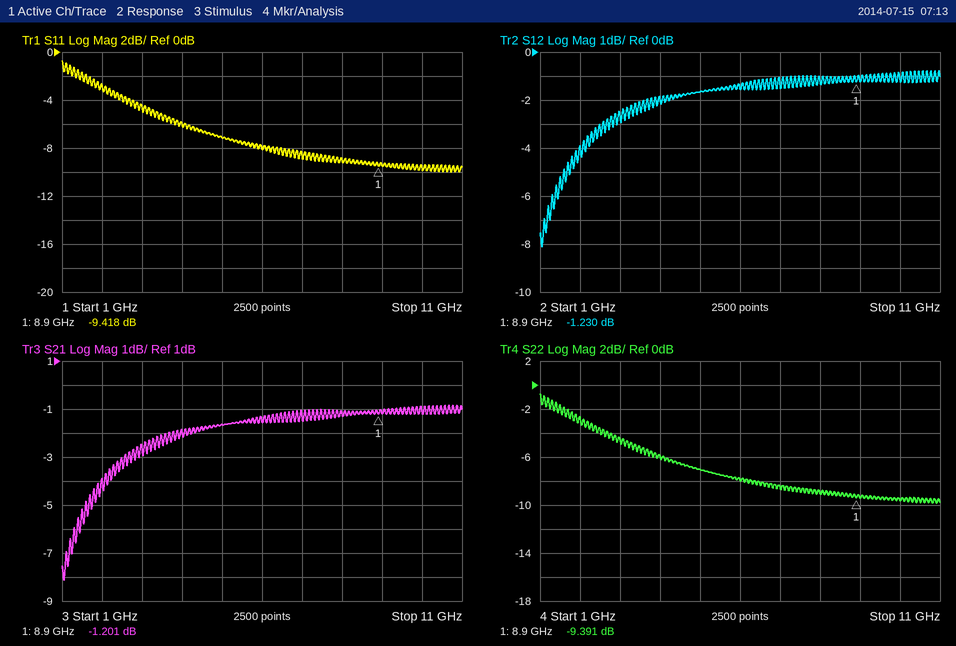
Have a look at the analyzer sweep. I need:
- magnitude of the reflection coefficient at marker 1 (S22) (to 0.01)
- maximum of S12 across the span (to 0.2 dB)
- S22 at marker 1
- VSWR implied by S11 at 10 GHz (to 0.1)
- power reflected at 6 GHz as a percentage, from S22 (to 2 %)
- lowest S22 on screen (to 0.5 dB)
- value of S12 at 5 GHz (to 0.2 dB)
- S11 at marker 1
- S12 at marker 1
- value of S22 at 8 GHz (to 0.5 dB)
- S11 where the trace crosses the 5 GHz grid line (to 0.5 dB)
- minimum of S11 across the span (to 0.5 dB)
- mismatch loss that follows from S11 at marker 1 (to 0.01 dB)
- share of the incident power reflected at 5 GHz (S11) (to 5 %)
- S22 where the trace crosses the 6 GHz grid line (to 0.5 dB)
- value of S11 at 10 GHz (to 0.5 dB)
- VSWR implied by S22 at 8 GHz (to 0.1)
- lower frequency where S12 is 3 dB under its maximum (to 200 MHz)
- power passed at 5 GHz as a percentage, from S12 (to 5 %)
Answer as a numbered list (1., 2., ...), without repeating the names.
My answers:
1. 0.34
2. -0.8 dB
3. -9.391 dB
4. 2.0
5. 16 %
6. -10.0 dB
7. -1.6 dB
8. -9.418 dB
9. -1.230 dB
10. -9.0 dB
11. -7.0 dB
12. -10.0 dB
13. 0.53 dB
14. 20 %
15. -8.0 dB
16. -9.5 dB
17. 2.1
18. 2.2 GHz
19. 70 %
